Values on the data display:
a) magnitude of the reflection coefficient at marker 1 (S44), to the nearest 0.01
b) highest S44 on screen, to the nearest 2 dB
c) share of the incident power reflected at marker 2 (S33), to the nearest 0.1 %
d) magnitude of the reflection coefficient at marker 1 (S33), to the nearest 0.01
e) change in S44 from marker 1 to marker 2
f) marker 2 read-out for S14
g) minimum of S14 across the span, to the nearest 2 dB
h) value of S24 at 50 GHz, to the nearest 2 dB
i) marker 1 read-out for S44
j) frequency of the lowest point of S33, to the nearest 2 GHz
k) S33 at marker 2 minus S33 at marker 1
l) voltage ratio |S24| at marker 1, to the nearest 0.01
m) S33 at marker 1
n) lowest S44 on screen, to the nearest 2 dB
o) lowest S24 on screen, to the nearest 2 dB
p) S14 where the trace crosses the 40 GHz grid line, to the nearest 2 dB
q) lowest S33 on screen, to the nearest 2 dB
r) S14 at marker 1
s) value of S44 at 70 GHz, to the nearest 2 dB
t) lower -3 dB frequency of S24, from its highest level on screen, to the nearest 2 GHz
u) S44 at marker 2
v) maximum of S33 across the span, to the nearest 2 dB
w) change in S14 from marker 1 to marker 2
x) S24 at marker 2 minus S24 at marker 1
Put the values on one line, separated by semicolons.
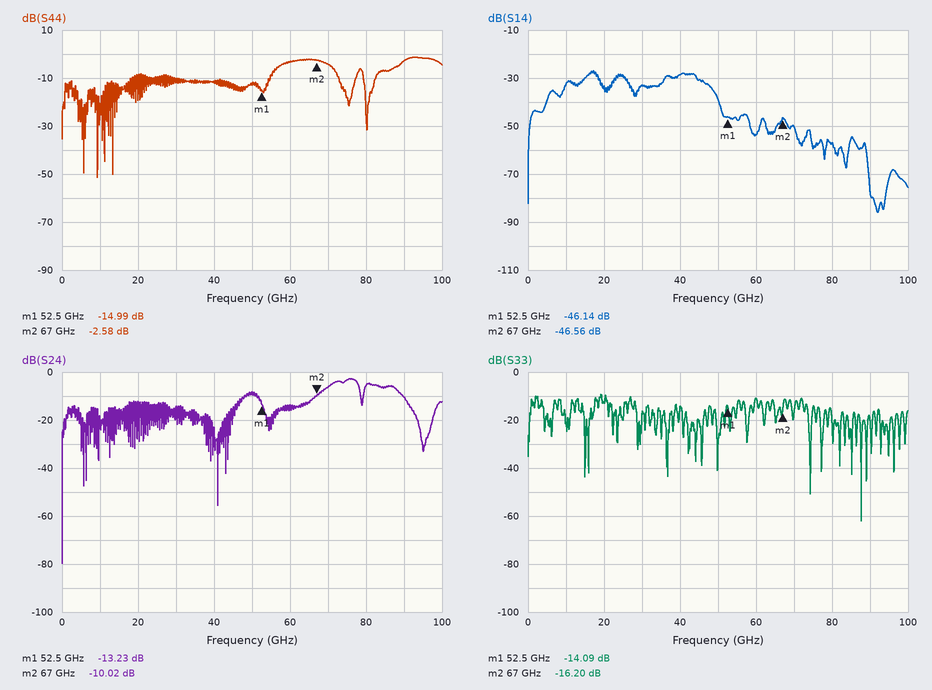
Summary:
0.18; -2 dB; 2.4 %; 0.20; 12.41 dB; -46.56 dB; -86 dB; -8 dB; -14.99 dB; 88 GHz; -2.11 dB; 0.22; -14.09 dB; -52 dB; -80 dB; -28 dB; -62 dB; -46.14 dB; -4 dB; 70 GHz; -2.58 dB; -10 dB; -0.42 dB; 3.21 dB
